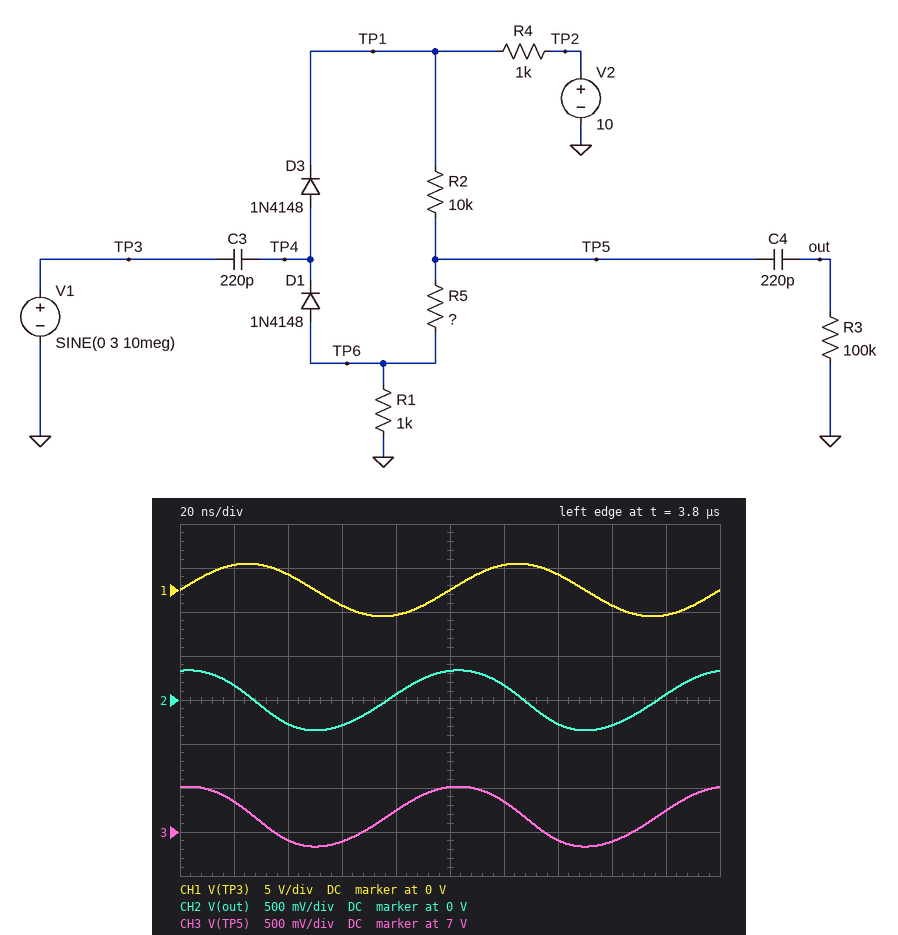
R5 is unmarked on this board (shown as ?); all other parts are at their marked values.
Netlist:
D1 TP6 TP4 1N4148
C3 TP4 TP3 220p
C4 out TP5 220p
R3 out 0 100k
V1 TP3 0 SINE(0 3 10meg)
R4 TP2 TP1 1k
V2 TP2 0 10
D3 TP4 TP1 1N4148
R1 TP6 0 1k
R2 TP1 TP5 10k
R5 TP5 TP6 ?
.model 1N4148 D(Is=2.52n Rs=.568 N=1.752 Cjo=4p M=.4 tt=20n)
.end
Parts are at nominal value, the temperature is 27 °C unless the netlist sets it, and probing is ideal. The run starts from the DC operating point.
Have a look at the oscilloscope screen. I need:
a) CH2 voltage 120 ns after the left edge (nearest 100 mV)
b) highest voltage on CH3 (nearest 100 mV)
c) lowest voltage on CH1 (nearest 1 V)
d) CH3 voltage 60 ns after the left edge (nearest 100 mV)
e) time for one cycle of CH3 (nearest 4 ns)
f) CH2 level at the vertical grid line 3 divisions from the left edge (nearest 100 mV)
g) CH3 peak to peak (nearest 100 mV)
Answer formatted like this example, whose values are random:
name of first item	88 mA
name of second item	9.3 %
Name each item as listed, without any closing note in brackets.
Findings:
CH2 voltage 120 ns after the left edge	200 mV
highest voltage on CH3	7.5 V
lowest voltage on CH1	-3 V
CH3 voltage 60 ns after the left edge	6.9 V
time for one cycle of CH3	100 ns
CH2 level at the vertical grid line 3 divisions from the left edge	-300 mV
CH3 peak to peak	700 mV
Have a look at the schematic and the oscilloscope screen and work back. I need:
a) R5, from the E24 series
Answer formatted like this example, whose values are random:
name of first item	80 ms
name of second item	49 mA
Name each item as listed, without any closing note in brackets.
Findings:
R5, from the E24 series	27 kΩ
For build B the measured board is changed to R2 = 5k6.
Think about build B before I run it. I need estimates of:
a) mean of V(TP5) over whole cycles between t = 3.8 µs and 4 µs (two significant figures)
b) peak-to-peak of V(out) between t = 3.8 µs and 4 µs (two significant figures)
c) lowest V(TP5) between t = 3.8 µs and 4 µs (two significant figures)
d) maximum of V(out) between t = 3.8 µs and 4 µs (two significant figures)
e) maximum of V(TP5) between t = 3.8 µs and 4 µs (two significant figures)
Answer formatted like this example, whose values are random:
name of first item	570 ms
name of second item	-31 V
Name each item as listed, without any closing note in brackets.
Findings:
mean of V(TP5) over whole cycles between t = 3.8 µs and 4 µs	8.1 V
peak-to-peak of V(out) between t = 3.8 µs and 4 µs	700 mV
lowest V(TP5) between t = 3.8 µs and 4 µs	7.7 V
maximum of V(out) between t = 3.8 µs and 4 µs	350 mV
maximum of V(TP5) between t = 3.8 µs and 4 µs	8.4 V
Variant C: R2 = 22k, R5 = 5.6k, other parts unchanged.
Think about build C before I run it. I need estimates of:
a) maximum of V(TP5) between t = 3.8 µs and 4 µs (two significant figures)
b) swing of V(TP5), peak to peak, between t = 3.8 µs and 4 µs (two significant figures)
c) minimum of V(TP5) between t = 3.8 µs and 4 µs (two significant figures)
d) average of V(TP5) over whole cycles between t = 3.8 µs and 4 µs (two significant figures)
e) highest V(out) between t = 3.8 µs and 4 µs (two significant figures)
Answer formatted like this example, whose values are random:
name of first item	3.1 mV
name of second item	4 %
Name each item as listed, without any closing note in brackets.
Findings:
maximum of V(TP5) between t = 3.8 µs and 4 µs	2.6 V
swing of V(TP5), peak to peak, between t = 3.8 µs and 4 µs	710 mV
minimum of V(TP5) between t = 3.8 µs and 4 µs	1.9 V
average of V(TP5) over whole cycles between t = 3.8 µs and 4 µs	2.2 V
highest V(out) between t = 3.8 µs and 4 µs	360 mV
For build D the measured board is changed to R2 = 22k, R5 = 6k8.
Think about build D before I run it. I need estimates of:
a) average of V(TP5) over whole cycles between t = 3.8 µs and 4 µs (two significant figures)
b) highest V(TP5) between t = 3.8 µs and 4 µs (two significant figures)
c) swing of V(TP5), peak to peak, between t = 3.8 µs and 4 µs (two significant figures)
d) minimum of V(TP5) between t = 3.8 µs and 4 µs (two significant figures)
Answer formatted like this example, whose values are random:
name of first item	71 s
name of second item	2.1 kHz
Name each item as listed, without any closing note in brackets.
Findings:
average of V(TP5) over whole cycles between t = 3.8 µs and 4 µs	2.5 V
highest V(TP5) between t = 3.8 µs and 4 µs	2.9 V
swing of V(TP5), peak to peak, between t = 3.8 µs and 4 µs	700 mV
minimum of V(TP5) between t = 3.8 µs and 4 µs	2.2 V
